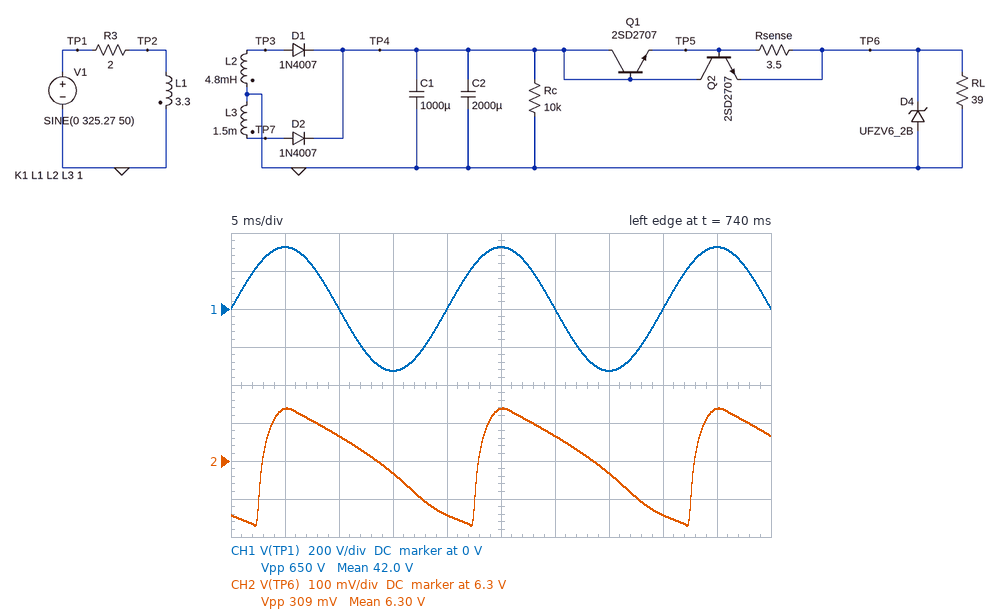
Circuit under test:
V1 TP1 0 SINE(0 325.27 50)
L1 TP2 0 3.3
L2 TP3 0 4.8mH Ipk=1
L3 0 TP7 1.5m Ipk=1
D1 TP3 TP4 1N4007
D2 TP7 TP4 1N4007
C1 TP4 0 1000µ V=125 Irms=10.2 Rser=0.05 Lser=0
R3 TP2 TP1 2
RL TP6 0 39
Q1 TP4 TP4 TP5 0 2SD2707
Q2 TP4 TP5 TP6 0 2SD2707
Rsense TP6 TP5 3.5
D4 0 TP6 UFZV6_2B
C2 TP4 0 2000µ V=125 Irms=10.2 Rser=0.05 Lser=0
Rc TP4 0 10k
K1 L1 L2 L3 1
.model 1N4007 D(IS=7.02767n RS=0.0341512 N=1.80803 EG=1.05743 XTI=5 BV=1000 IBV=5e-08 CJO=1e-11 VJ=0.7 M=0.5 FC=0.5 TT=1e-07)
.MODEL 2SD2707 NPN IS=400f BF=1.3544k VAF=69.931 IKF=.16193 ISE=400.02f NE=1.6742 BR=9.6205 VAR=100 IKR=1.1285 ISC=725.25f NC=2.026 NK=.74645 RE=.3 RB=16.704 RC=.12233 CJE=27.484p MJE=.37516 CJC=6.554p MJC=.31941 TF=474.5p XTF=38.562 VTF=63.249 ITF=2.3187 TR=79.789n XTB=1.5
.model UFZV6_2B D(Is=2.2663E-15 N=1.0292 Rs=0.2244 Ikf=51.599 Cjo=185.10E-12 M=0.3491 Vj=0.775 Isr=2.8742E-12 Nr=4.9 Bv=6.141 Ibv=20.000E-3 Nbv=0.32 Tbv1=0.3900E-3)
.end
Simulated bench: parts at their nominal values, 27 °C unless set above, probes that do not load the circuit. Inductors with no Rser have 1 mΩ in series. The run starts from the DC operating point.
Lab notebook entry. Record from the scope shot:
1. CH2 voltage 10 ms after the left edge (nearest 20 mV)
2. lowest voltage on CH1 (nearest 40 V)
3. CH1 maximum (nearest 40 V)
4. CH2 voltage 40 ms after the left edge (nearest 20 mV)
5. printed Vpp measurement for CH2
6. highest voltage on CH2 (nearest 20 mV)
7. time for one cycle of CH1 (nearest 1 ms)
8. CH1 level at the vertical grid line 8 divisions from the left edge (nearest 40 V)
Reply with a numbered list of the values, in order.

1. 6.36 V
2. -320 V
3. 320 V
4. 6.16 V
5. 309 mV
6. 6.44 V
7. 20 ms
8. 0 V
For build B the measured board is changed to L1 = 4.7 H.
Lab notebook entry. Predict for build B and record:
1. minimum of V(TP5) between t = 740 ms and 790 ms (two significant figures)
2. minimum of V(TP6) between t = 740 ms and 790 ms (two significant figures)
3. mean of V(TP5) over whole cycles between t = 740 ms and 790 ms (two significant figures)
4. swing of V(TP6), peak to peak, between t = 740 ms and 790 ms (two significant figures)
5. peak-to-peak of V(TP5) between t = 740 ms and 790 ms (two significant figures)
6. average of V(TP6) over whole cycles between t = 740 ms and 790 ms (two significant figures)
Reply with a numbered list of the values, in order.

1. 6.4 V
2. 5.9 V
3. 7.0 V
4. 470 mV
5. 1.5 V
6. 6.2 V
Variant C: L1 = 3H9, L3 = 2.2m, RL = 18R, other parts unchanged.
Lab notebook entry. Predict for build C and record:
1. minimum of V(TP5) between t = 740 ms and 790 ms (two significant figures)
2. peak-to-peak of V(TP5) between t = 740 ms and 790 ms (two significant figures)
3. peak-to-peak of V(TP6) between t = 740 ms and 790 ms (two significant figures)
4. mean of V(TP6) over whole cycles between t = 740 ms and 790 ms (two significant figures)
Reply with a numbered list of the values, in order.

1. 6.2 V
2. 2.2 V
3. 910 mV
4. 6.1 V
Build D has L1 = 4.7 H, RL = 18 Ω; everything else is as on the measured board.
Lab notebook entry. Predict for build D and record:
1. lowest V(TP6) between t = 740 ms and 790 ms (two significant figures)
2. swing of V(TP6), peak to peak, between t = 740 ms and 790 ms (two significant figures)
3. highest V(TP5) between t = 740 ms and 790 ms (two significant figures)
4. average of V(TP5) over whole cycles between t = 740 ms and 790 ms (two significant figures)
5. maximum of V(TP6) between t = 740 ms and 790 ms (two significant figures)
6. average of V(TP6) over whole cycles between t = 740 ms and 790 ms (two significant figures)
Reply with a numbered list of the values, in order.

1. 5.2 V
2. 1.1 V
3. 7.9 V
4. 6.9 V
5. 6.3 V
6. 5.9 V
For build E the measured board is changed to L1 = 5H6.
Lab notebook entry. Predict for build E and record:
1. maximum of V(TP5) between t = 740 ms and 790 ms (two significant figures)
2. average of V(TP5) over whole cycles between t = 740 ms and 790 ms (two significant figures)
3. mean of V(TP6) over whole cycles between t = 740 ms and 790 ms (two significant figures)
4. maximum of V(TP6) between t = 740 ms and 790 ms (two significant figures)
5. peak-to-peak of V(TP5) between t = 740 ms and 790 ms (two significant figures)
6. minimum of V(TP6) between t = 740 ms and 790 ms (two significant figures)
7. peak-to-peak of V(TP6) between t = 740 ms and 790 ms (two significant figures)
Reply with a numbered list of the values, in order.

1. 7.5 V
2. 6.8 V
3. 6.1 V
4. 6.3 V
5. 1.2 V
6. 5.7 V
7. 560 mV
